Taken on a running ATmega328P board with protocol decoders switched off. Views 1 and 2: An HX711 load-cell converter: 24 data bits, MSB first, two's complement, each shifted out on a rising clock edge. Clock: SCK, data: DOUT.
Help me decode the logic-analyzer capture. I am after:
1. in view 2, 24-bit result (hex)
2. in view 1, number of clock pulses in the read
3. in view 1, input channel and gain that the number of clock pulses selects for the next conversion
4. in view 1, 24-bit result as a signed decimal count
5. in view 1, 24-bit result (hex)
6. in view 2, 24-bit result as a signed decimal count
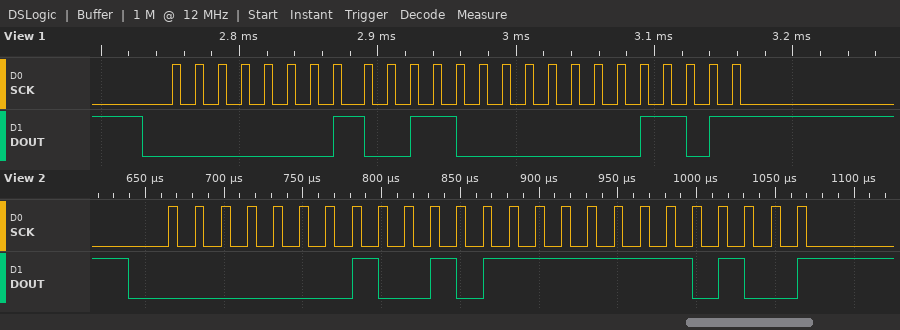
0x012FF4
25
channel A, gain 128
77837
0x01300D
77812
